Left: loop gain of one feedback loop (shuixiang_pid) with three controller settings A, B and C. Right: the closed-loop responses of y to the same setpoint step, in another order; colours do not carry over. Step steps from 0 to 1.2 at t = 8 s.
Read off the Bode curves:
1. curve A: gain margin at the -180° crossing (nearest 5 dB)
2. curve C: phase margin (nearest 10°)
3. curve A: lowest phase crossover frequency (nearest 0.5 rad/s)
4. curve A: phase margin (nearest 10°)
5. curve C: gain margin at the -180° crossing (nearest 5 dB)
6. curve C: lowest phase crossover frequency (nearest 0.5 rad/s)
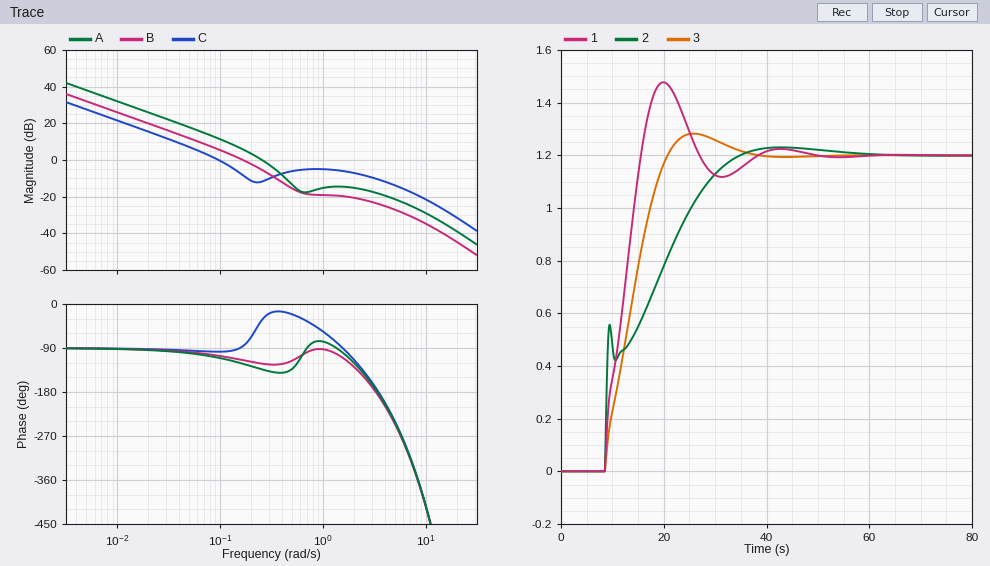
20 dB
80°
3.5 rad/s
50°
10 dB
3.5 rad/s
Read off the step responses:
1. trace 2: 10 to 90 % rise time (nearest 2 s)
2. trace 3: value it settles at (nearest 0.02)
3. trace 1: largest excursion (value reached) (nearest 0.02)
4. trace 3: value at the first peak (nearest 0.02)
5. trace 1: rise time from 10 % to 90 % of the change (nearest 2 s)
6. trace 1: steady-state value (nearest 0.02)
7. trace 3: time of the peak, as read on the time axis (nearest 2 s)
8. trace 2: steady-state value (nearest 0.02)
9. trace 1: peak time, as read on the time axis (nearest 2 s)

20 s
1.20
1.48
1.28
6 s
1.20
26 s
1.20
20 s
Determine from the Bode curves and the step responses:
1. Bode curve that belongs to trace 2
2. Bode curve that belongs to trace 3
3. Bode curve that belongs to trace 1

C
B
A
